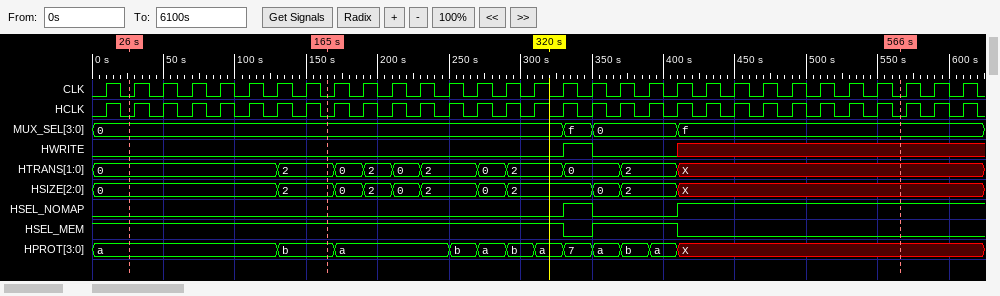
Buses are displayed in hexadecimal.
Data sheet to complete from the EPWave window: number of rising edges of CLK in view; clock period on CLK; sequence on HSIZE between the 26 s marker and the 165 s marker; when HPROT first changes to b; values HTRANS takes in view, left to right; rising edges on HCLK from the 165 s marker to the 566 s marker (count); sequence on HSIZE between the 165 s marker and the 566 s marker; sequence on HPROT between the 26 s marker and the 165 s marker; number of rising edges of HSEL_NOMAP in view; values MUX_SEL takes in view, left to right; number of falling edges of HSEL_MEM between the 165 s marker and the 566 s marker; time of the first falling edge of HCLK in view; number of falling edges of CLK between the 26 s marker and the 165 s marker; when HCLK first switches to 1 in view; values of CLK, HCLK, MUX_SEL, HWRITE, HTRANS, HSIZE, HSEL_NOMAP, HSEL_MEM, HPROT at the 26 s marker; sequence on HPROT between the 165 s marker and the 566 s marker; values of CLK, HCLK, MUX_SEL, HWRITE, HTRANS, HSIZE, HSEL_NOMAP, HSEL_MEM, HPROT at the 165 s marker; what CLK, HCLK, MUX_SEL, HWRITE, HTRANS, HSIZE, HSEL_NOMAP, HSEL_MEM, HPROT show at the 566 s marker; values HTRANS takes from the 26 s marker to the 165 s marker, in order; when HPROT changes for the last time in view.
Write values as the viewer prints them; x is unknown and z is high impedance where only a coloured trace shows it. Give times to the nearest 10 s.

31
20 s
0, 2
130 s
0, 2, 0, 2, 0, 2, 0, 2, 0, 2, X
20
2, 0, 2, 0, 2, 0, 2, 0, 2, X
a, b
2
0, f, 0, f
2
20 s
7
10 s
CLK=0, HCLK=0, MUX_SEL=0, HWRITE=0, HTRANS=0, HSIZE=0, HSEL_NOMAP=0, HSEL_MEM=1, HPROT=a
b, a, b, a, b, a, 7, a, b, a, X
CLK=0, HCLK=0, MUX_SEL=0, HWRITE=0, HTRANS=2, HSIZE=2, HSEL_NOMAP=0, HSEL_MEM=1, HPROT=b
CLK=0, HCLK=0, MUX_SEL=f, HWRITE=x, HTRANS=X, HSIZE=X, HSEL_NOMAP=1, HSEL_MEM=0, HPROT=X
0, 2
410 s
